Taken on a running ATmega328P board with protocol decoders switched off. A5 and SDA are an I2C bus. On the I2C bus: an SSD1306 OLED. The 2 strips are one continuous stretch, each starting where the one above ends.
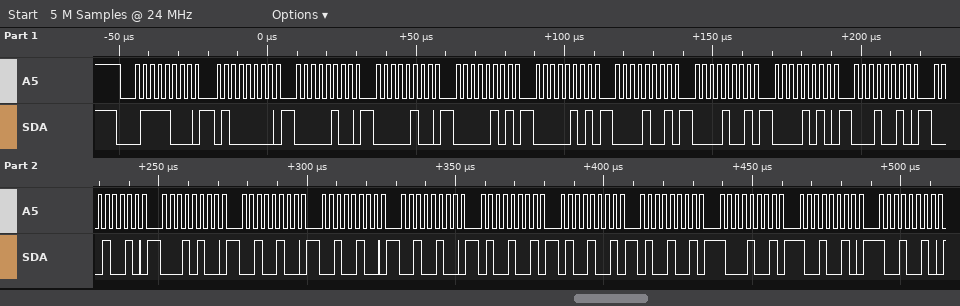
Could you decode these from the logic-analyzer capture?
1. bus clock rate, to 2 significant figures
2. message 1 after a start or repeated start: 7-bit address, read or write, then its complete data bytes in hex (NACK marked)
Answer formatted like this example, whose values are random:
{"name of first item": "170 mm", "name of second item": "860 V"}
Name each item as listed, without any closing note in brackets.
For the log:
{"bus clock rate, to 2 significant figures": "400 kHz", "message 1 after a start or repeated start: 7-bit address, read or write, then its complete data bytes in hex": "0x3C write: 40 04 04 05 05 09 09 0A 12 12 14 24 24 24 49 49 49 89 92 92"}
